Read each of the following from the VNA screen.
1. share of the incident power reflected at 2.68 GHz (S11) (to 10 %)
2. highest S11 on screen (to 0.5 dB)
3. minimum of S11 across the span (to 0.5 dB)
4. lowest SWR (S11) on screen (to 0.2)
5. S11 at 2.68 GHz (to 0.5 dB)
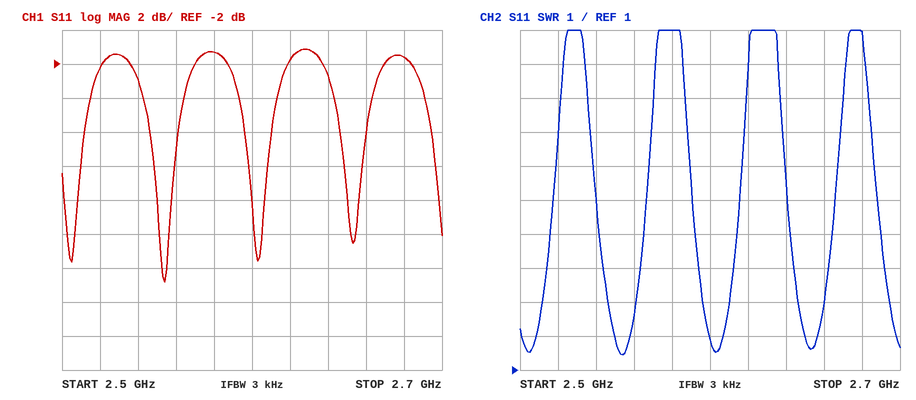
70 %
-1.0 dB
-15.0 dB
1.4
-1.5 dB
